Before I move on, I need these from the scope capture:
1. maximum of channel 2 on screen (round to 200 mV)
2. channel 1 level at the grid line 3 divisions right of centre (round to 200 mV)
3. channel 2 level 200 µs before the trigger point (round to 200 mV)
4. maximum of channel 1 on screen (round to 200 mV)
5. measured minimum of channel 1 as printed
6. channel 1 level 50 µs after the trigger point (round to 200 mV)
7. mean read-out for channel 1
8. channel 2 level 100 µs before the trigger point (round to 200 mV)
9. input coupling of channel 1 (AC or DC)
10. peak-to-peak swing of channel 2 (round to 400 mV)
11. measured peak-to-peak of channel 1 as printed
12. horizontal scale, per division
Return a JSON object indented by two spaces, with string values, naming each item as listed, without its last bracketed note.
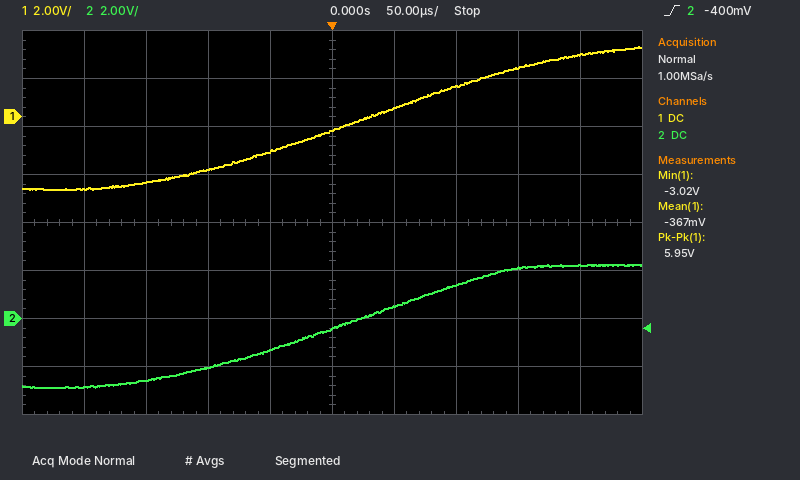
{
  "maximum of channel 2 on screen": "2.2 V",
  "channel 1 level at the grid line 3 divisions right of centre": "2.0 V",
  "channel 2 level 200 µs before the trigger point": "-2.8 V",
  "maximum of channel 1 on screen": "3.0 V",
  "measured minimum of channel 1 as printed": "-3.02 V",
  "channel 1 level 50 µs after the trigger point": "400 mV",
  "mean read-out for channel 1": "-367 mV",
  "channel 2 level 100 µs before the trigger point": "-2.0 V",
  "input coupling of channel 1": "DC",
  "peak-to-peak swing of channel 2": "5.2 V",
  "measured peak-to-peak of channel 1 as printed": "5.95 V",
  "horizontal scale, per division": "50 µs"
}
